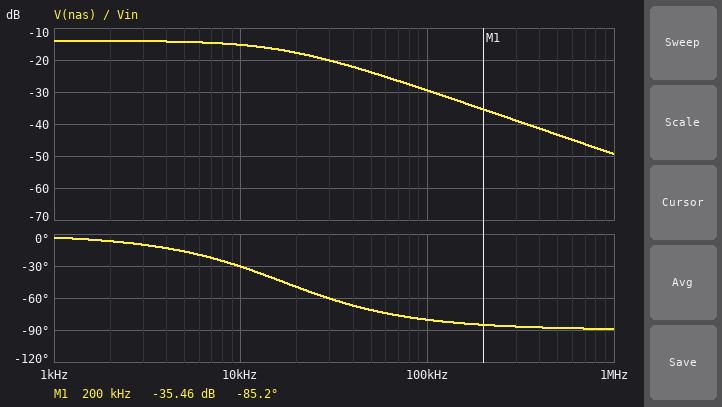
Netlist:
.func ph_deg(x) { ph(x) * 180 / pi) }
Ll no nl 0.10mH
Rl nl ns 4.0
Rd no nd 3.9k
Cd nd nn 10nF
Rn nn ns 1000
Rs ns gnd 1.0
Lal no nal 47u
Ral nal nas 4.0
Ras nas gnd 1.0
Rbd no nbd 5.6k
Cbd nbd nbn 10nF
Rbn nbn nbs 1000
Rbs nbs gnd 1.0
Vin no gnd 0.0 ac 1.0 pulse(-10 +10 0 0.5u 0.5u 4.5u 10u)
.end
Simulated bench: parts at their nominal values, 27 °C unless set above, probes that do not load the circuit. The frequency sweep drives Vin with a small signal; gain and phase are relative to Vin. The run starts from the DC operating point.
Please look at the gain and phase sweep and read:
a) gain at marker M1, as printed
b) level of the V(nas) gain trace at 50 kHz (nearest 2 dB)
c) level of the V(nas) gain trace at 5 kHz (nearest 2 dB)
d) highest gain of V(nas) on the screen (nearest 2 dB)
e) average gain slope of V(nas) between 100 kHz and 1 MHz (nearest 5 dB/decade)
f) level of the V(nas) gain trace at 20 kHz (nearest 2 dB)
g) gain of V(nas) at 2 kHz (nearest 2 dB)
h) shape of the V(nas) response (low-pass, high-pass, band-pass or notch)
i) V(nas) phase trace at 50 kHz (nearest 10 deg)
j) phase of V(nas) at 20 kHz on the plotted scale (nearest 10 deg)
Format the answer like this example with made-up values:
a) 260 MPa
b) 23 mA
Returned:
a) -35.46 dB
b) -24 dB
c) -14 dB
d) -14 dB
e) -20 dB/decade
f) -18 dB
g) -14 dB
h) low-pass
i) -70 deg
j) -50 deg
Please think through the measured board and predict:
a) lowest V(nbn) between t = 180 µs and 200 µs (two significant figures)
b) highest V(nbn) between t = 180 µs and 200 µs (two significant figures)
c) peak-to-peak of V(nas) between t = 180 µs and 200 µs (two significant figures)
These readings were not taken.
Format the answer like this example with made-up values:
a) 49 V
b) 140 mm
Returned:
a) -1.5 V
b) 1.7 V
c) 990 mV
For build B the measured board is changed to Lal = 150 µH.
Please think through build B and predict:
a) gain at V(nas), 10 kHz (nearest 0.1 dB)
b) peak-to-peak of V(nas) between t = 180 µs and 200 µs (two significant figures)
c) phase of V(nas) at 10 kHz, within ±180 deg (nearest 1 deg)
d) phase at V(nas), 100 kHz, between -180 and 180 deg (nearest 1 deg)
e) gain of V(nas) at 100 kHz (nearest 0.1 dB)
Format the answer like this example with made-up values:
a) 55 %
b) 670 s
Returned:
a) -20.6 dB
b) 320 mV
c) -62 deg
d) -87 deg
e) -39.5 dB
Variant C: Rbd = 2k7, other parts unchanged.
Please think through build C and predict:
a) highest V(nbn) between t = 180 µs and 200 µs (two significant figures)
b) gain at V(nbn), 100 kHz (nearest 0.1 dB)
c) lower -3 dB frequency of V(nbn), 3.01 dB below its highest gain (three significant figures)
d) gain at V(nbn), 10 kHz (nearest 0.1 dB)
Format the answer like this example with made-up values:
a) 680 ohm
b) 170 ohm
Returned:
a) 2.9 V
b) -11.4 dB
c) 4.30 kHz
d) -12.1 dB
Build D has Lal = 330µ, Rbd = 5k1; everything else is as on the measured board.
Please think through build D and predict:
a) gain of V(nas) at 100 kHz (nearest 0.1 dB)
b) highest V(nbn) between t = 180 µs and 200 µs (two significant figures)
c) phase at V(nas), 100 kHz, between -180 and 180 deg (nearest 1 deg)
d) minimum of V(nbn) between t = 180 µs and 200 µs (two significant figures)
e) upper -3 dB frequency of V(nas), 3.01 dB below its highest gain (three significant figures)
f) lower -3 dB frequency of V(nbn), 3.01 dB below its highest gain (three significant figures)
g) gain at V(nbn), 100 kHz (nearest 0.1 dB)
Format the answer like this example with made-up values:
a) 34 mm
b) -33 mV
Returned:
a) -46.3 dB
b) 1.8 V
c) -89 deg
d) -1.6 V
e) 2.41 kHz
f) 2.61 kHz
g) -15.7 dB
